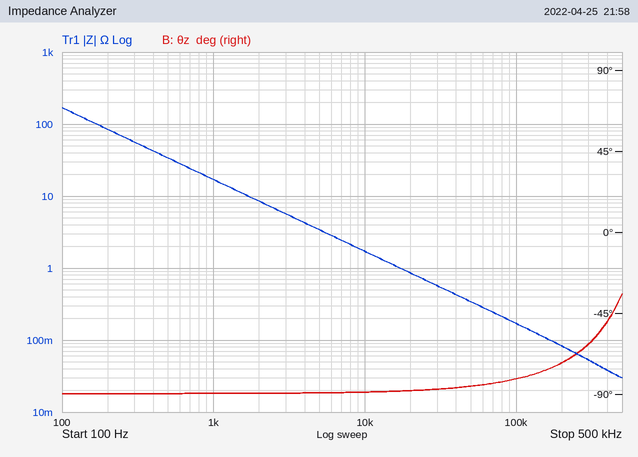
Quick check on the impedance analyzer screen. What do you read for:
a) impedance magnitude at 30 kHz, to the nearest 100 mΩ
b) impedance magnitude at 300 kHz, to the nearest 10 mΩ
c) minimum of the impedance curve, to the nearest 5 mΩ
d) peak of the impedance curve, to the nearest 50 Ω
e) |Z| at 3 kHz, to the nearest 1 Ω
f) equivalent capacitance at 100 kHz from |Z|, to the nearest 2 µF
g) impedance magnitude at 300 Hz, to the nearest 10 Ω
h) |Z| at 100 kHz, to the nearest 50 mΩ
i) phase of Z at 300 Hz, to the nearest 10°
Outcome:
600 mΩ
50 mΩ
30 mΩ
150 Ω
6 Ω
10 µF
60 Ω
150 mΩ
-90°
